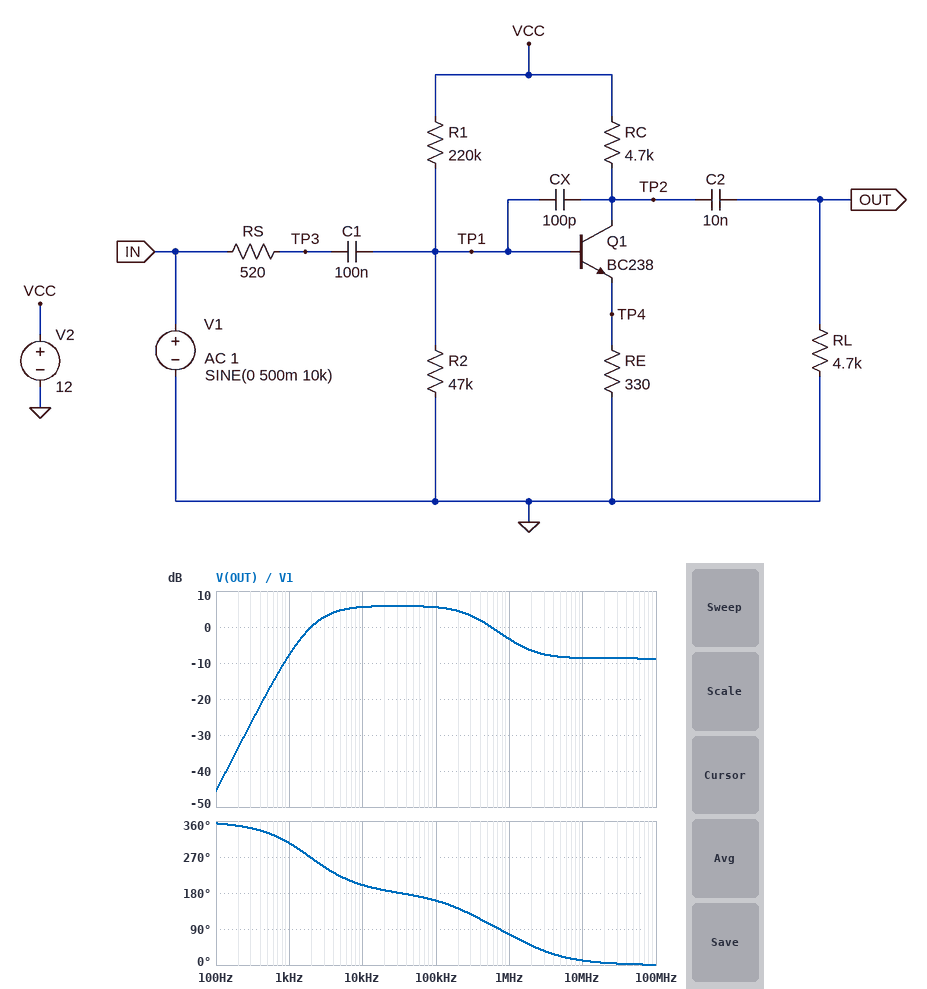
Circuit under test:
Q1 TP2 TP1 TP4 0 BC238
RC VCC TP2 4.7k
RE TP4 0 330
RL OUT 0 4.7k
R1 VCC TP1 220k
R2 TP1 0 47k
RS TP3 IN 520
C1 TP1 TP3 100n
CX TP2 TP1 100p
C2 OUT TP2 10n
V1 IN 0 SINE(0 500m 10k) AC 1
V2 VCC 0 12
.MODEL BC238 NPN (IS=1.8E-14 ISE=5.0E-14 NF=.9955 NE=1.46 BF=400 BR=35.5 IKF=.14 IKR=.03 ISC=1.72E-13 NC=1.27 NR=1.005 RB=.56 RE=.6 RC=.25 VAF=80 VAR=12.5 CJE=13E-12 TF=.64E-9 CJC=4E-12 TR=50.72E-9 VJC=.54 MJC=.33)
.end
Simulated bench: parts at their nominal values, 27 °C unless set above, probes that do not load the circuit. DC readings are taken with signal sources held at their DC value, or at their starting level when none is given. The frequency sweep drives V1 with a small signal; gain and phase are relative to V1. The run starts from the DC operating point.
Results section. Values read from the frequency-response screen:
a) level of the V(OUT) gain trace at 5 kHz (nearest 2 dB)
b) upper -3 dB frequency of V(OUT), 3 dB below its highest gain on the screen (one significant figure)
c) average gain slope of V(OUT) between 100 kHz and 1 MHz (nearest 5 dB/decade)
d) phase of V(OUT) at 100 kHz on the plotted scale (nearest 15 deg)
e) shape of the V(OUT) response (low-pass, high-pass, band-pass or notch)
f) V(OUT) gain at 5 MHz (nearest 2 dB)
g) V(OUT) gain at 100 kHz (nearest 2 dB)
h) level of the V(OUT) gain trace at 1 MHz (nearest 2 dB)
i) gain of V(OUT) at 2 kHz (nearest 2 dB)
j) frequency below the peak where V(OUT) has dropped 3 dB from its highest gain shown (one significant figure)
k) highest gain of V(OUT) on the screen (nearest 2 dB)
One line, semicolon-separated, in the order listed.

4 dB; 300 kHz; -10 dB/decade; 165 deg; band-pass; -8 dB; 6 dB; -4 dB; 0 dB; 3 kHz; 6 dB
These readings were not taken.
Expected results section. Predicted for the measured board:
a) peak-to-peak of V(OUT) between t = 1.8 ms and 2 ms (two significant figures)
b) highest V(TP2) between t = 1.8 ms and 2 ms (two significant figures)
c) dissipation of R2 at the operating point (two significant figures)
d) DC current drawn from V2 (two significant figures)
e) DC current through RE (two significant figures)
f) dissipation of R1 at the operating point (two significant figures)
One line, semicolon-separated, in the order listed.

6.1 V; 7.0 V; 45 µW; 2.4 mA; 2.4 mA; 510 µW
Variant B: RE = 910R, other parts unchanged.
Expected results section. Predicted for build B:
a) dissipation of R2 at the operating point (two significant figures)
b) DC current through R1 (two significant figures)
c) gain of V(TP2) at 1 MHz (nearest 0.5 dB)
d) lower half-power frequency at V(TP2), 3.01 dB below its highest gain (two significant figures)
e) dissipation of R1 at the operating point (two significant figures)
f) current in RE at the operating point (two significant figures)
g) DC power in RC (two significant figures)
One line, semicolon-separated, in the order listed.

79 µW; 46 µA; 0 dB; 44 Hz; 460 µW; 1.4 mA; 9.2 mW
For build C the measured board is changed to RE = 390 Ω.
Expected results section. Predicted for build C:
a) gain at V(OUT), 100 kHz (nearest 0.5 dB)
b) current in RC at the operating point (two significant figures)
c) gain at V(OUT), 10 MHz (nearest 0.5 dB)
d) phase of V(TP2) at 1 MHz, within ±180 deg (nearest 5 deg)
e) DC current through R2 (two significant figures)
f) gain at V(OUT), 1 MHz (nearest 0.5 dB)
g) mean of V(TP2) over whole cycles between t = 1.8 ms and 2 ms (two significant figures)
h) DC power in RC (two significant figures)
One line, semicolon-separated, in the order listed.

7.5 dB; 2.3 mA; -8.0 dB; 80 deg; 34 µA; -1.5 dB; 3.6 V; 26 mW
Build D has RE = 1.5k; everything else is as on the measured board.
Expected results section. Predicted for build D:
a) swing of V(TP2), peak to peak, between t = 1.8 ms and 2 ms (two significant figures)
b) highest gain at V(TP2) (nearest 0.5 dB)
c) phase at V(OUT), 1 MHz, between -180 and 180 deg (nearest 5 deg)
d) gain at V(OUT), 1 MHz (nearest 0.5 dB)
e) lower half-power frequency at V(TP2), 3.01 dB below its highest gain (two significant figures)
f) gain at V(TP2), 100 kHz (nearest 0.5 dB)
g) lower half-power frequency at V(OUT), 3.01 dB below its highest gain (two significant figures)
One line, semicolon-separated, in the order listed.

1.6 V; 9.5 dB; 70 deg; -1.5 dB; 42 Hz; 3.5 dB; 1.7 kHz
